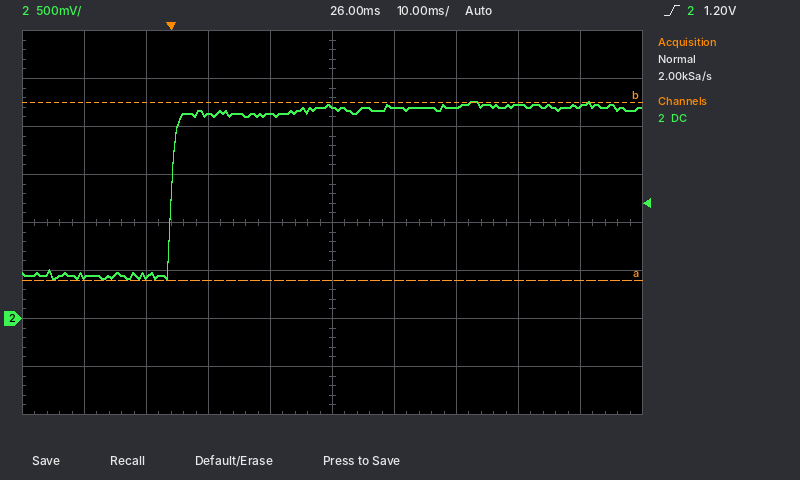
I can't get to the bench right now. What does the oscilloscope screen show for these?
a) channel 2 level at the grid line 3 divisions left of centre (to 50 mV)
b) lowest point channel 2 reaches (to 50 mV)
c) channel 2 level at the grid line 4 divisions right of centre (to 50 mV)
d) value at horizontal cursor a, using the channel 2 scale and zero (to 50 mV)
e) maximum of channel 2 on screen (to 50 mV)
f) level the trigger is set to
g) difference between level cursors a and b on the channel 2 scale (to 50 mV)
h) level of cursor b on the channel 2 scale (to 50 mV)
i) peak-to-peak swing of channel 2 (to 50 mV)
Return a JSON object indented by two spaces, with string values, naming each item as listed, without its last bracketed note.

{
  "channel 2 level at the grid line 3 divisions left of centre": "450 mV",
  "lowest point channel 2 reaches": "400 mV",
  "channel 2 level at the grid line 4 divisions right of centre": "2.20 V",
  "value at horizontal cursor a, using the channel 2 scale and zero": "400 mV",
  "maximum of channel 2 on screen": "2.25 V",
  "level the trigger is set to": "1.20 V",
  "difference between level cursors a and b on the channel 2 scale": "1.85 V",
  "level of cursor b on the channel 2 scale": "2.25 V",
  "peak-to-peak swing of channel 2": "1.85 V"
}
